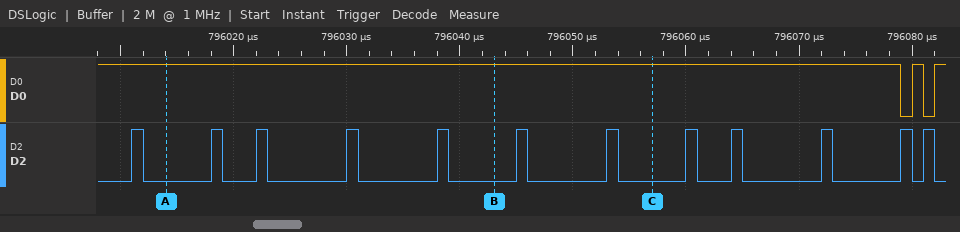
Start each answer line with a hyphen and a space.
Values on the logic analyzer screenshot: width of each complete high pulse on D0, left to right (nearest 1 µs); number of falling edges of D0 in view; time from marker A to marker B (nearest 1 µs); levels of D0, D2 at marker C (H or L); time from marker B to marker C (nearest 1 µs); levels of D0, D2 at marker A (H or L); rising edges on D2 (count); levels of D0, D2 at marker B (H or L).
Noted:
- 1 µs
- 2
- 29 µs
- D0=H, D2=L
- 14 µs
- D0=H, D2=L
- 12
- D0=H, D2=L
